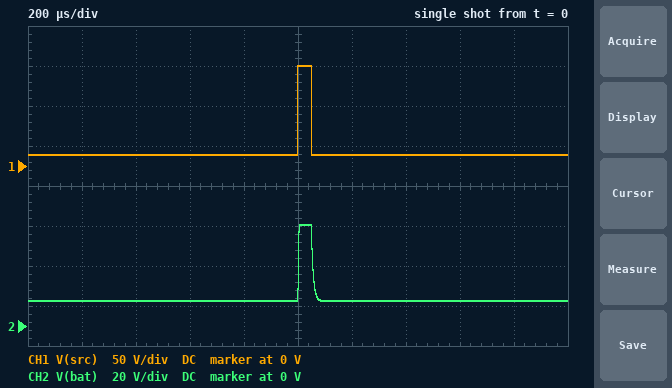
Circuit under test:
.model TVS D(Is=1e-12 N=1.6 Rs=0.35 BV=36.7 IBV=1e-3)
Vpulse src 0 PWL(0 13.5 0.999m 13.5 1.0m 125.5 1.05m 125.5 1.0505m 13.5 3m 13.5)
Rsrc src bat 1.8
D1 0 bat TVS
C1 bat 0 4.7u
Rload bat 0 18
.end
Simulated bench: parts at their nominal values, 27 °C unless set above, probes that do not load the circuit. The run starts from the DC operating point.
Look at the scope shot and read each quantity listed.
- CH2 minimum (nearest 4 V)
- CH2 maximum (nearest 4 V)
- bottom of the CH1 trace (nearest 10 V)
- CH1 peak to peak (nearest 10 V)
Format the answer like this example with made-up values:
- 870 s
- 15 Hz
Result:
- 12 V
- 52 V
- 10 V
- 110 V
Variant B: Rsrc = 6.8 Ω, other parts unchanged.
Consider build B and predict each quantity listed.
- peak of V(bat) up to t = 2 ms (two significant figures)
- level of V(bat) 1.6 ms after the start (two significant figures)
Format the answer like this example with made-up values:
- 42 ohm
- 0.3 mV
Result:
- 41 V
- 9.8 V
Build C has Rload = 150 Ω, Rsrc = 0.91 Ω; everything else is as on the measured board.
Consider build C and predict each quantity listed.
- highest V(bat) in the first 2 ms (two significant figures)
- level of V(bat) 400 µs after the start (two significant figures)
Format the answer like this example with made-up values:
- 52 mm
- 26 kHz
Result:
- 62 V
- 13 V
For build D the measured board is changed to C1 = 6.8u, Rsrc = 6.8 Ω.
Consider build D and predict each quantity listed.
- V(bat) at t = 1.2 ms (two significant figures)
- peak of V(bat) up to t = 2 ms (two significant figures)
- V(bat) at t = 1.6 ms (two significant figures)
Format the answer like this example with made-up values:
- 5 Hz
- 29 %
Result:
- 10 V
- 41 V
- 9.8 V
